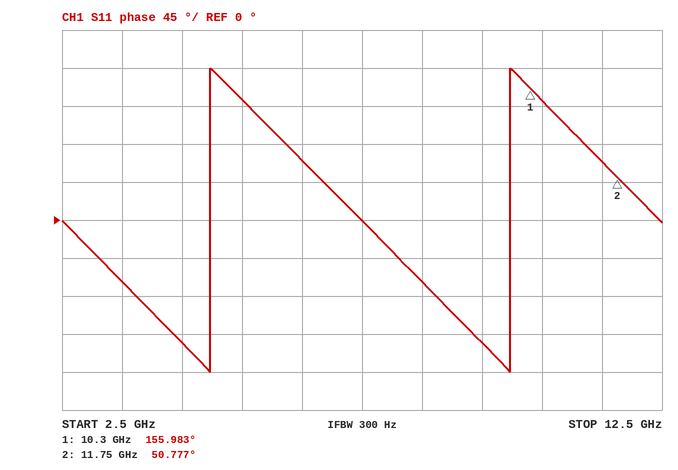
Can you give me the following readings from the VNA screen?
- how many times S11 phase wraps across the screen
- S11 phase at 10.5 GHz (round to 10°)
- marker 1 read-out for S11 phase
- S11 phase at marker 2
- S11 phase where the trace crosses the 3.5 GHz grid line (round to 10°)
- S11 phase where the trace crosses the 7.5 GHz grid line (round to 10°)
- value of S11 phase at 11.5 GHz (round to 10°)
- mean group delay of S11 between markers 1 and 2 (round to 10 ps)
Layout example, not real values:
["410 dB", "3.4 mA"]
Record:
["2", "140°", "155.983°", "50.777°", "-70°", "0°", "70°", "200 ps"]
